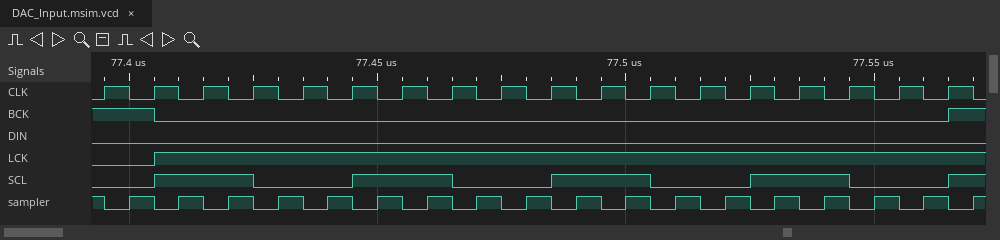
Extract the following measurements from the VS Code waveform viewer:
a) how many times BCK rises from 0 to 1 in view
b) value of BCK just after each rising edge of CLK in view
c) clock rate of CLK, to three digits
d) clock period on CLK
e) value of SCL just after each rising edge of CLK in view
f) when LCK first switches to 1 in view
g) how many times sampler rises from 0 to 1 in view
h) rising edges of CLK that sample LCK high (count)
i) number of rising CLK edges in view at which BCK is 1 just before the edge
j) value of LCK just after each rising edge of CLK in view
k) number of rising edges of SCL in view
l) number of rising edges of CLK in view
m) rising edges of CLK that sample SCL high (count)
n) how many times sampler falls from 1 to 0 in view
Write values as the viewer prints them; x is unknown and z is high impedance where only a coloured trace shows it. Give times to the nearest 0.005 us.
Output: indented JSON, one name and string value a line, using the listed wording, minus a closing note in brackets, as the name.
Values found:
{
  "how many times BCK rises from 0 to 1 in view": "1",
  "value of BCK just after each rising edge of CLK in view": "1 0 0 0 0 0 0 0 0 0 0 0 0 0 0 0 0 1",
  "clock rate of CLK, to three digits": "100 MHz",
  "clock period on CLK": "0.01 us",
  "value of SCL just after each rising edge of CLK in view": "0 1 1 0 0 1 1 0 0 1 1 0 0 1 1 0 0 1",
  "when LCK first switches to 1 in view": "77.405 us",
  "how many times sampler rises from 0 to 1 in view": "18",
  "rising edges of CLK that sample LCK high": "16",
  "number of rising CLK edges in view at which BCK is 1 just before the edge": "2",
  "value of LCK just after each rising edge of CLK in view": "0 1 1 1 1 1 1 1 1 1 1 1 1 1 1 1 1 1",
  "number of rising edges of SCL in view": "5",
  "number of rising edges of CLK in view": "18",
  "rising edges of CLK that sample SCL high": "8",
  "how many times sampler falls from 1 to 0 in view": "18"
}
